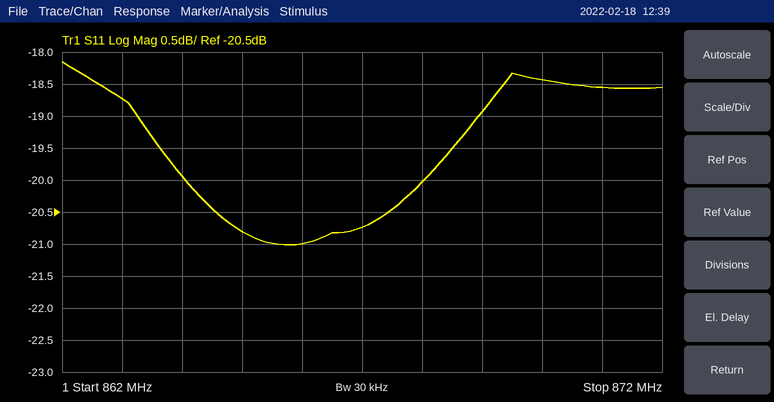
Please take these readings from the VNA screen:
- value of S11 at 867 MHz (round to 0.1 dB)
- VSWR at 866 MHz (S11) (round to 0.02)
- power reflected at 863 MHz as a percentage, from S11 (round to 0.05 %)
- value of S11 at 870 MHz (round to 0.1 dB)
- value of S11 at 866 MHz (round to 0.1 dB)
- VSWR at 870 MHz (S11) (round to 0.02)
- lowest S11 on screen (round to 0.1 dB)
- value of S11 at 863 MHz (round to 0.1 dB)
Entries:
-20.7 dB
1.20
1.35 %
-18.4 dB
-21.0 dB
1.28
-21.0 dB
-18.7 dB
